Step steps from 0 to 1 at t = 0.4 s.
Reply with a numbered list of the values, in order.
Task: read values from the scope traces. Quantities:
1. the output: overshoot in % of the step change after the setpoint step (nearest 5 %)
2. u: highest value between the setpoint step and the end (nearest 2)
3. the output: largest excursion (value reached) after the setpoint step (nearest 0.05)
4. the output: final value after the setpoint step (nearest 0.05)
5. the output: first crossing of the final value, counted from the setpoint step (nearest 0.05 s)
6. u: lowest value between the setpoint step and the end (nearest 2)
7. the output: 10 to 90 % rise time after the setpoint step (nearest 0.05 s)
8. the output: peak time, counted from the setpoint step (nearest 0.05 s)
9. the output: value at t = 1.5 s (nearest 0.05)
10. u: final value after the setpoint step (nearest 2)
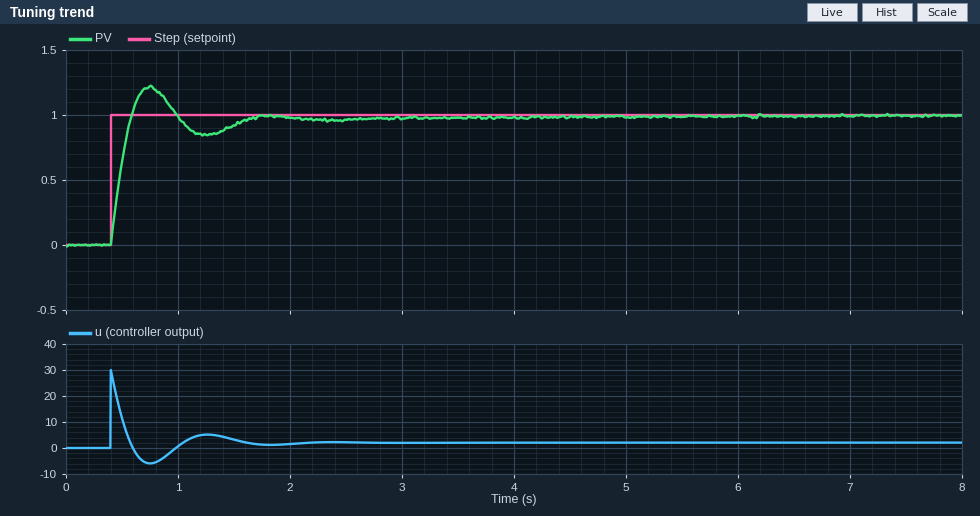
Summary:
1. 20 %
2. 30
3. 1.20
4. 1.00
5. 0.20 s
6. -6
7. 0.15 s
8. 0.35 s
9. 0.90
10. 2
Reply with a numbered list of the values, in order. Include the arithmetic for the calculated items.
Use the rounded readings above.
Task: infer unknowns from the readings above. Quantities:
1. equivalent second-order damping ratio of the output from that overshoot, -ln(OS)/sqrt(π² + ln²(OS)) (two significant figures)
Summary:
1. ln(0.2) = -1.609; 1.609 / sqrt(9.870 + 2.590) = 0.46
